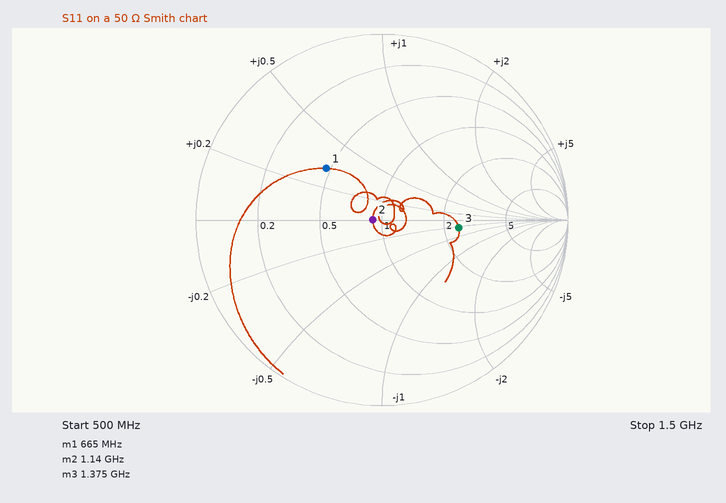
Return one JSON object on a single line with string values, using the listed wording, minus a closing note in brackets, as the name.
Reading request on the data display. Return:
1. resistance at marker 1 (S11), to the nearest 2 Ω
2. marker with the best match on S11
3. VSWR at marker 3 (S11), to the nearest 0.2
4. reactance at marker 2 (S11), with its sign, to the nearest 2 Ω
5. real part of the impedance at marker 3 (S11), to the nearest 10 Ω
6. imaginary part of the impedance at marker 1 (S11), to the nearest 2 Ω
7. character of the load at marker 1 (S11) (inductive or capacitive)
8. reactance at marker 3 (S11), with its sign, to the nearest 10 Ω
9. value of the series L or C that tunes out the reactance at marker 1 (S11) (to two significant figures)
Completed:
{"resistance at marker 1 (S11), to the nearest 2 Ω": "24 Ω", "marker with the best match on S11": "marker 2", "VSWR at marker 3 (S11), to the nearest 0.2": "2.4", "reactance at marker 2 (S11), with its sign, to the nearest 2 Ω": "0 Ω", "real part of the impedance at marker 3 (S11), to the nearest 10 Ω": "120 Ω", "imaginary part of the impedance at marker 1 (S11), to the nearest 2 Ω": "+16 Ω", "character of the load at marker 1 (S11)": "inductive", "reactance at marker 3 (S11), with its sign, to the nearest 10 Ω": "-10 Ω", "value of the series L or C that tunes out the reactance at marker 1 (S11)": "15 pF"}
